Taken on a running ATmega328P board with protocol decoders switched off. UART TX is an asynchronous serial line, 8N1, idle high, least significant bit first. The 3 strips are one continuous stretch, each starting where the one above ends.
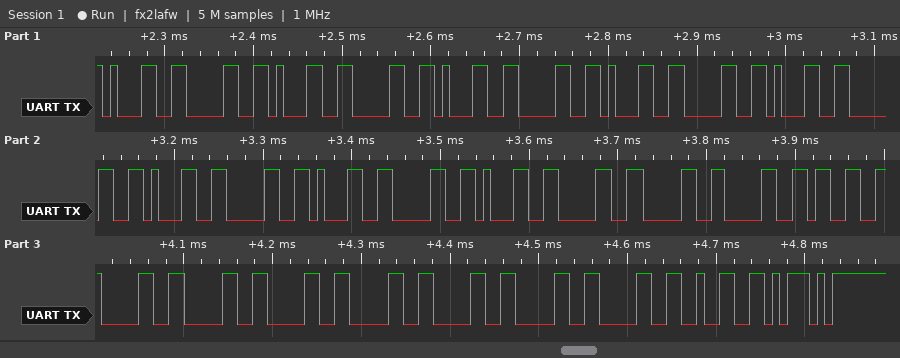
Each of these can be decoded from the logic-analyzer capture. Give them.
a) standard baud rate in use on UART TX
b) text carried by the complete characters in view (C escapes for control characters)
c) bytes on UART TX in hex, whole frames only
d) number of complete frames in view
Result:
115200 baud
"101010101010101000300000002]"
31 30 31 30 31 30 31 30 31 30 31 30 31 30 31 30 30 30 33 30 30 30 30 30 30 30 32 5D
28
